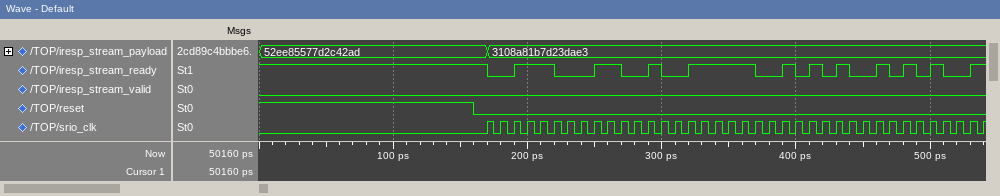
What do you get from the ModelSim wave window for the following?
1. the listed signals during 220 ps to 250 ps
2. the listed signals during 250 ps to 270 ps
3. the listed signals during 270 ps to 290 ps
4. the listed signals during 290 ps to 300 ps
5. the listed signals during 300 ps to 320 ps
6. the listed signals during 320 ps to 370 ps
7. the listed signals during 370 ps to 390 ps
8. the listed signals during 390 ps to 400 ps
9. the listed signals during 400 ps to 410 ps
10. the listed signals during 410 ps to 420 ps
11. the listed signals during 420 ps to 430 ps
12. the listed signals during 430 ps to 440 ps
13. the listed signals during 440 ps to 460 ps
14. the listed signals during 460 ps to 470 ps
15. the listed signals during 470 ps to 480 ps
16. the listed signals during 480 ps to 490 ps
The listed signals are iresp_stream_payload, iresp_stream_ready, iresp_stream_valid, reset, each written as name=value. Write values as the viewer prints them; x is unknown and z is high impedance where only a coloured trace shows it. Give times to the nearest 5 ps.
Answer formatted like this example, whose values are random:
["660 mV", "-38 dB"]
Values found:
["iresp_stream_payload=3108a81b7d23dae3, iresp_stream_ready=0, iresp_stream_valid=0, reset=0", "iresp_stream_payload=3108a81b7d23dae3, iresp_stream_ready=1, iresp_stream_valid=0, reset=0", "iresp_stream_payload=3108a81b7d23dae3, iresp_stream_ready=0, iresp_stream_valid=0, reset=0", "iresp_stream_payload=3108a81b7d23dae3, iresp_stream_ready=1, iresp_stream_valid=0, reset=0", "iresp_stream_payload=3108a81b7d23dae3, iresp_stream_ready=0, iresp_stream_valid=0, reset=0", "iresp_stream_payload=3108a81b7d23dae3, iresp_stream_ready=1, iresp_stream_valid=0, reset=0", "iresp_stream_payload=3108a81b7d23dae3, iresp_stream_ready=0, iresp_stream_valid=0, reset=0", "iresp_stream_payload=3108a81b7d23dae3, iresp_stream_ready=1, iresp_stream_valid=0, reset=0", "iresp_stream_payload=3108a81b7d23dae3, iresp_stream_ready=0, iresp_stream_valid=0, reset=0", "iresp_stream_payload=3108a81b7d23dae3, iresp_stream_ready=1, iresp_stream_valid=0, reset=0", "iresp_stream_payload=3108a81b7d23dae3, iresp_stream_ready=0, iresp_stream_valid=0, reset=0", "iresp_stream_payload=3108a81b7d23dae3, iresp_stream_ready=1, iresp_stream_valid=0, reset=0", "iresp_stream_payload=3108a81b7d23dae3, iresp_stream_ready=0, iresp_stream_valid=0, reset=0", "iresp_stream_payload=3108a81b7d23dae3, iresp_stream_ready=1, iresp_stream_valid=0, reset=0", "iresp_stream_payload=3108a81b7d23dae3, iresp_stream_ready=0, iresp_stream_valid=0, reset=0", "iresp_stream_payload=3108a81b7d23dae3, iresp_stream_ready=1, iresp_stream_valid=0, reset=0"]
